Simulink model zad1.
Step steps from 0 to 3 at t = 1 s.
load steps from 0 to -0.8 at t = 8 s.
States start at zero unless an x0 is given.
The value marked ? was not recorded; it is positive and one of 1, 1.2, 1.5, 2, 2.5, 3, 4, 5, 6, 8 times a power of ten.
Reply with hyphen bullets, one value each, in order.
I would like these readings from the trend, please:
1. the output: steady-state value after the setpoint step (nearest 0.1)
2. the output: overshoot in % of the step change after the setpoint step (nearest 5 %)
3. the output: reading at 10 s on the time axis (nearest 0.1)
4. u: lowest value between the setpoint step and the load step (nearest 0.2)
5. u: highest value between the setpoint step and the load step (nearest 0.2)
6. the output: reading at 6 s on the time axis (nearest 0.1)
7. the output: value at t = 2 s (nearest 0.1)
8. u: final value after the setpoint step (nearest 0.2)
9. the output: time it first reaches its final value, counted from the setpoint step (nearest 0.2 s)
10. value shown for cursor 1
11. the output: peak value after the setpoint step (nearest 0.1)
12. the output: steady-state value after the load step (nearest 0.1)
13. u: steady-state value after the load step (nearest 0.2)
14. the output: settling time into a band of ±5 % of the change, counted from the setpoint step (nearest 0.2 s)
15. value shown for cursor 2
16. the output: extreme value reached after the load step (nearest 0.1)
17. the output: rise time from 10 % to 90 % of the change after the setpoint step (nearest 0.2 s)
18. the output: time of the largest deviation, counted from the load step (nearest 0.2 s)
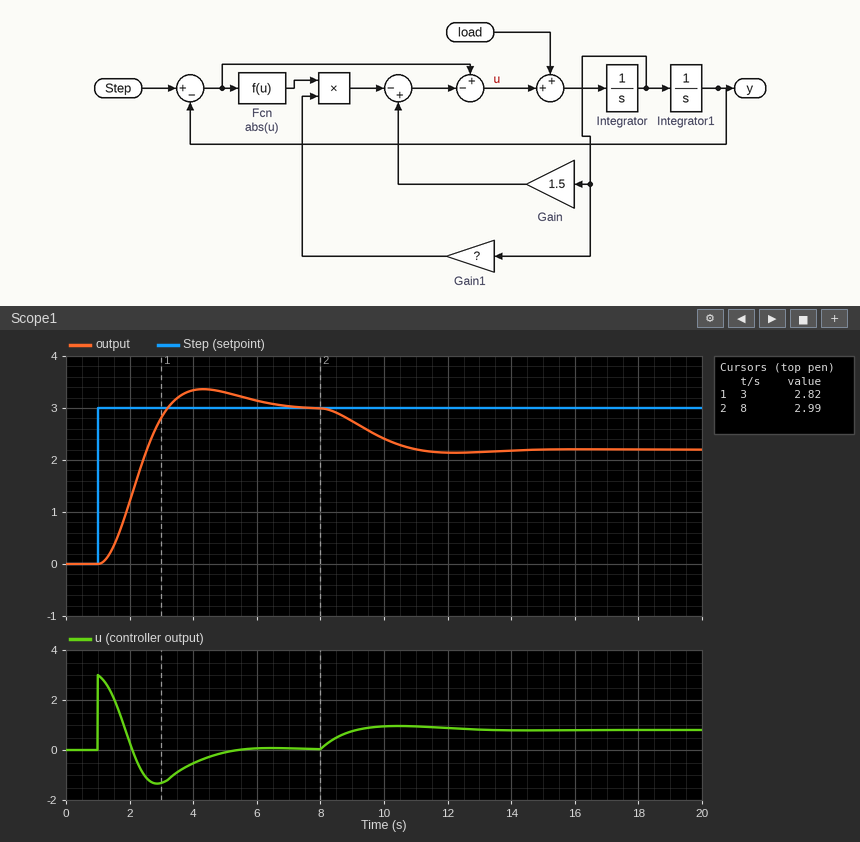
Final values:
- 3.0
- 10 %
- 2.4
- -1.4
- 3.0
- 3.1
- 1.2
- 0.0
- 2.2 s
- 2.82
- 3.4
- 2.2
- 0.8
- 5.0 s
- 2.99
- 2.1
- 1.4 s
- 4.2 s
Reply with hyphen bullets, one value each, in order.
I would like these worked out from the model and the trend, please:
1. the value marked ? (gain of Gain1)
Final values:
- 0.4
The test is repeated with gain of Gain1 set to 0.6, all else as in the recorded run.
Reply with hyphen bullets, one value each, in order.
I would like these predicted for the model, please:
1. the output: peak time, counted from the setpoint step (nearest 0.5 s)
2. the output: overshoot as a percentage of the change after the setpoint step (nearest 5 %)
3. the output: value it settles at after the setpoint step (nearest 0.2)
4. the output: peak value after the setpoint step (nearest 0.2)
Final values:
- 3.0 s
- 20 %
- 3.0
- 3.6
